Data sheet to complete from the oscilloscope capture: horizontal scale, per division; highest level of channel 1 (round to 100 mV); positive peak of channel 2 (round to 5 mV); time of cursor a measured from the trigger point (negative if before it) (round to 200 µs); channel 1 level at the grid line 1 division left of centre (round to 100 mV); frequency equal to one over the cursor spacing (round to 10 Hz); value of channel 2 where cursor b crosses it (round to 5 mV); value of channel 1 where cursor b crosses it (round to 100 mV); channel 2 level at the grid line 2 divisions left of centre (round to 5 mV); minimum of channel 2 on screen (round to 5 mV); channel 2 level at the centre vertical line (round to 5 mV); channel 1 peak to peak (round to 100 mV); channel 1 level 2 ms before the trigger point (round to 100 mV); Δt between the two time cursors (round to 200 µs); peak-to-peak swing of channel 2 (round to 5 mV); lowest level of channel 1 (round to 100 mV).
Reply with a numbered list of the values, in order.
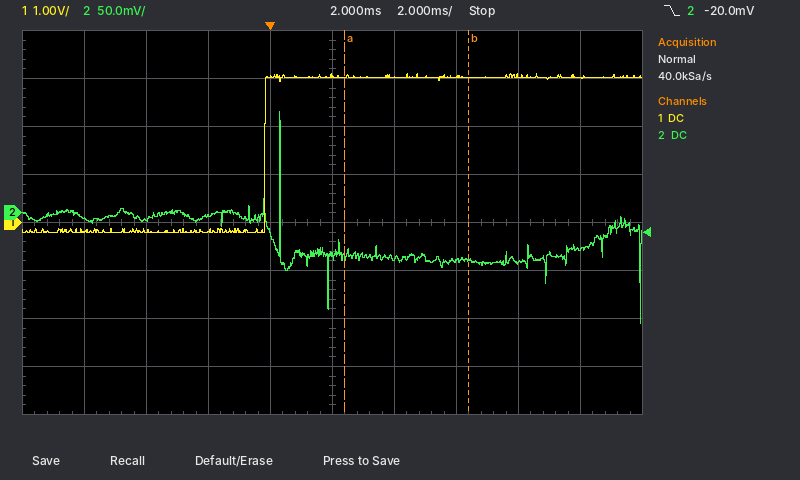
1. 2 ms
2. 3.1 V
3. 105 mV
4. +2.4 ms
5. 3.0 V
6. 250 Hz
7. -50 mV
8. 3.0 V
9. -5 mV
10. -115 mV
11. -45 mV
12. 3.3 V
13. -200 mV
14. 4.0 ms
15. 220 mV
16. -200 mV
